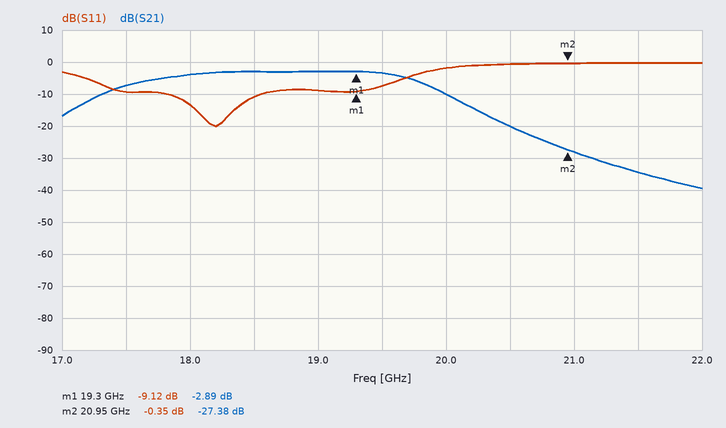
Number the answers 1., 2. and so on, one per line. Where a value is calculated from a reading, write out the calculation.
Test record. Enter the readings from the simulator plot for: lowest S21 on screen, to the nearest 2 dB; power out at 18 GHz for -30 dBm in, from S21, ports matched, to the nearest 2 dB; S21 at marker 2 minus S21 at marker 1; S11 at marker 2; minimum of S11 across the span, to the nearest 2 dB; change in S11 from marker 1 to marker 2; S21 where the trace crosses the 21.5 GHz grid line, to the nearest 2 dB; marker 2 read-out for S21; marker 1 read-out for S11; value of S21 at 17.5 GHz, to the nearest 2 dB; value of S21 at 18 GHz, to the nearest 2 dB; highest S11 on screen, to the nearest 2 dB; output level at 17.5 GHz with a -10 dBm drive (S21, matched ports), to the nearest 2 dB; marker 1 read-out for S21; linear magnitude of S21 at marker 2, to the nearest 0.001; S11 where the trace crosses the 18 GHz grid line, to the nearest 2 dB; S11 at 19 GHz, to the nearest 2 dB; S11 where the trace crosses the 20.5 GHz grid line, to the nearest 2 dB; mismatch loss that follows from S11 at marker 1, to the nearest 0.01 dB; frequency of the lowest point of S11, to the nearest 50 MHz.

1. -40 dB
2. -30 dBm + (-4 dB) = -34 dBm
3. -27.38 − (-2.89) = -24.49 dB
4. -0.35 dB
5. -20 dB
6. -0.35 − (-9.12) = 8.77 dB
7. -34 dB
8. -27.38 dB
9. -9.12 dB
10. -8 dB
11. -4 dB
12. 0 dB
13. -10 dBm + (-8 dB) = -18 dBm
14. -2.89 dB
15. 10^(-27.38/20) ≈ 0.043
16. -14 dB
17. -8 dB
18. 0 dB
19. −10 log10(1 − 10^(-9.12/10)) ≈ 0.57 dB
20. 18.20 GHz
